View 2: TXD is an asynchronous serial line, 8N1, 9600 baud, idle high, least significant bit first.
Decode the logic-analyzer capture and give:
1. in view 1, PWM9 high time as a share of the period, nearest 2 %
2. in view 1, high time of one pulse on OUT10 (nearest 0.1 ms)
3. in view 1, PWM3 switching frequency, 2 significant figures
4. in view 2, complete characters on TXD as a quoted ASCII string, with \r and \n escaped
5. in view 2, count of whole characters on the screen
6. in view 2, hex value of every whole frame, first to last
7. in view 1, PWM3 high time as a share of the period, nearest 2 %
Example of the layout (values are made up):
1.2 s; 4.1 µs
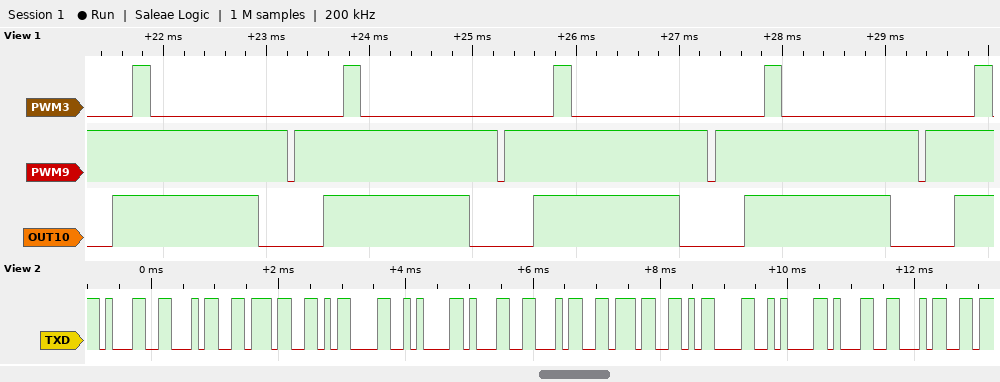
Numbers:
96 %; 1.4 ms; 490 Hz; "147\r\n147\r\n14"; 12; 31 34 37 0D 0A 31 34 37 0D 0A 31 34; 8 %
